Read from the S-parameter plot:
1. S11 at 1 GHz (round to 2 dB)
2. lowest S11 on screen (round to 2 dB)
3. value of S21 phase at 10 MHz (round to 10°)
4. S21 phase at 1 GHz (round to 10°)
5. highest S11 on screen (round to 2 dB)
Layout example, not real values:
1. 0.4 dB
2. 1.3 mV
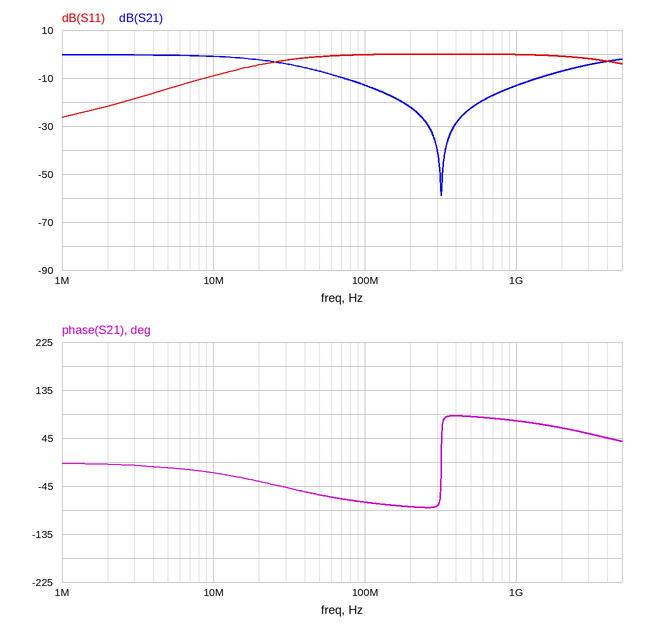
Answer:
1. 0 dB
2. -26 dB
3. -20°
4. 80°
5. 0 dB
